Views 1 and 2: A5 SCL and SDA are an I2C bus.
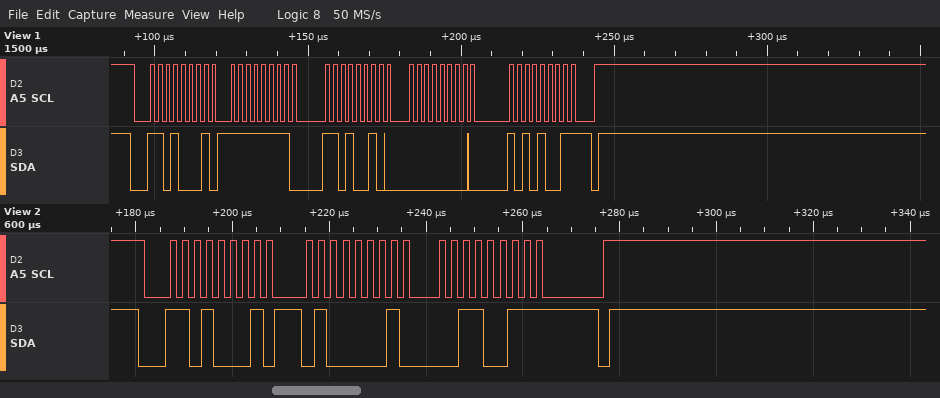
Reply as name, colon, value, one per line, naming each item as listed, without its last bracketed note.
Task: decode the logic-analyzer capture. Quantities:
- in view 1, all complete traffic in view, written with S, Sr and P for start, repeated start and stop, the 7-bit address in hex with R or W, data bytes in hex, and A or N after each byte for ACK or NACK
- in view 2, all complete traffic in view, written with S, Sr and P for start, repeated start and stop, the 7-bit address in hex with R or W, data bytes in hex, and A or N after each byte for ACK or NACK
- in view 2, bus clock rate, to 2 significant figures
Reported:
in view 1, all complete traffic in view, written with S, Sr and P for start, repeated start and stop, the 7-bit address in hex with R or W, data bytes in hex, and A or N after each byte for ACK or NACK: S 68R A FF A D2 A 00 A A9 N P
in view 2, all complete traffic in view, written with S, Sr and P for start, repeated start and stop, the 7-bit address in hex with R or W, data bytes in hex, and A or N after each byte for ACK or NACK: S 68R A 41 A 33 N P
in view 2, bus clock rate, to 2 significant figures: 400 kHz
